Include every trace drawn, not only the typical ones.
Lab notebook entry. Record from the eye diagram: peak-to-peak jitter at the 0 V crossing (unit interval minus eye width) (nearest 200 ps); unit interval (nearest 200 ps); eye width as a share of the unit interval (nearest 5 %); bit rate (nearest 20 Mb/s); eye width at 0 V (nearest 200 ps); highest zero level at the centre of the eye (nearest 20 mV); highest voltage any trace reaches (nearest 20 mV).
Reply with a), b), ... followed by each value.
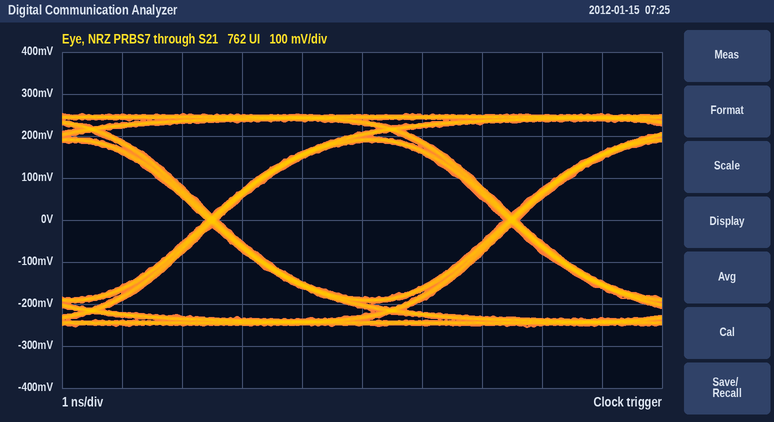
a) 200 ps
b) 5.0 ns
c) 95 %
d) 200 Mb/s
e) 4.8 ns
f) -180 mV
g) 260 mV
